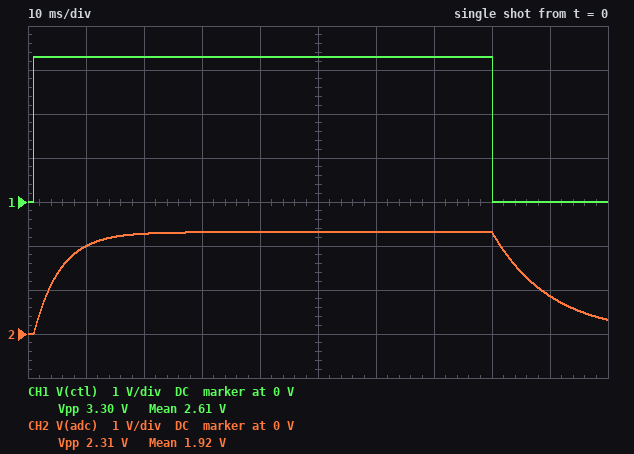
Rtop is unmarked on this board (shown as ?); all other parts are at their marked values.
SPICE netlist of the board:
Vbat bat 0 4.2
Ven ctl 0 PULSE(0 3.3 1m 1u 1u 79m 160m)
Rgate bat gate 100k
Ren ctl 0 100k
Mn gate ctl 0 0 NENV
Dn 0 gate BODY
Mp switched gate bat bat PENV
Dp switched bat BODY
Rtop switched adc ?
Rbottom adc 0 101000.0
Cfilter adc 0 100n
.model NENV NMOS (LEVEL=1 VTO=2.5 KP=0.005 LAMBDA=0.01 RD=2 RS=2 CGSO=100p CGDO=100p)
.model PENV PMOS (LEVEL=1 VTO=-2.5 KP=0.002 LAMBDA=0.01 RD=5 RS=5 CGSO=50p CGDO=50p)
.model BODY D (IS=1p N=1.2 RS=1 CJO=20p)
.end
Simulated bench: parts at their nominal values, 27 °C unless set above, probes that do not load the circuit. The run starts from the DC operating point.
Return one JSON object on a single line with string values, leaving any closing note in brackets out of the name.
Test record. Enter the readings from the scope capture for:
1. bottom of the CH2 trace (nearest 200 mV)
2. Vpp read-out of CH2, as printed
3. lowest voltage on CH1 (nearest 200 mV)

{"bottom of the CH2 trace": "0 V", "Vpp read-out of CH2, as printed": "2.31 V", "lowest voltage on CH1": "0 V"}
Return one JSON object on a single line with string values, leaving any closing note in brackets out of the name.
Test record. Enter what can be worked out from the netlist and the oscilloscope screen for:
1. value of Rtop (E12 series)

{"value of Rtop": "82 kΩ"}
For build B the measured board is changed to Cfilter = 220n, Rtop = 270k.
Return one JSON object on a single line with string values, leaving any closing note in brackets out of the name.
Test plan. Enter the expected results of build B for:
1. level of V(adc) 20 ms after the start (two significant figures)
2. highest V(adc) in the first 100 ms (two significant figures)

{"level of V(adc) 20 ms after the start": "790 mV", "highest V(adc) in the first 100 ms": "1.1 V"}
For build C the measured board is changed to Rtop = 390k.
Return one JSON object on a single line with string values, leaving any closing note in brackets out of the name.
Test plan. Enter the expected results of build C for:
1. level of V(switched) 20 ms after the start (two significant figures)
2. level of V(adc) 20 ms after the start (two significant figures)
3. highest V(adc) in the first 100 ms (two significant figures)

{"level of V(switched) 20 ms after the start": "4.2 V", "level of V(adc) 20 ms after the start": "780 mV", "highest V(adc) in the first 100 ms": "860 mV"}
